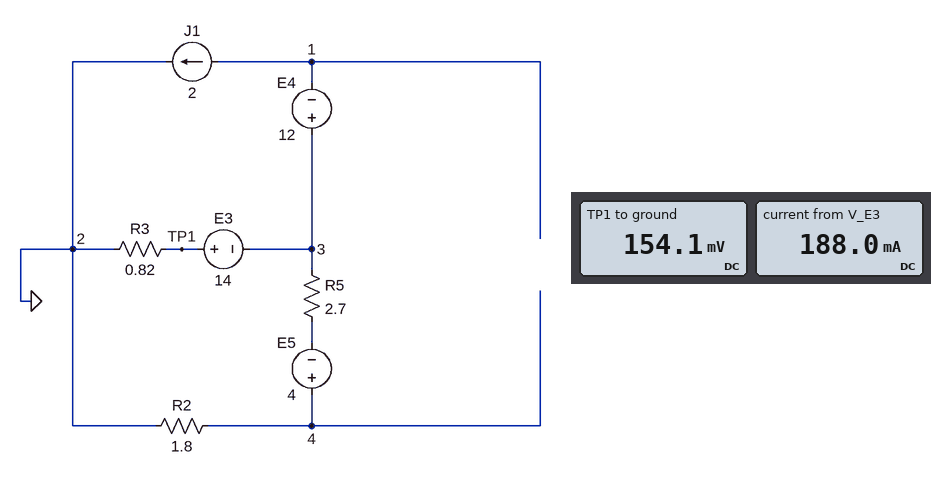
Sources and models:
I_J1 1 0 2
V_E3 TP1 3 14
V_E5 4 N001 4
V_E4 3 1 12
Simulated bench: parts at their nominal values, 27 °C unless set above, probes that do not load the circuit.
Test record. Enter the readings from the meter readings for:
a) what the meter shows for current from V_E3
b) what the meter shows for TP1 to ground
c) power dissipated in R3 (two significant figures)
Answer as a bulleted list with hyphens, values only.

- 188.0 mA
- 154.1 mV
- 29 mW
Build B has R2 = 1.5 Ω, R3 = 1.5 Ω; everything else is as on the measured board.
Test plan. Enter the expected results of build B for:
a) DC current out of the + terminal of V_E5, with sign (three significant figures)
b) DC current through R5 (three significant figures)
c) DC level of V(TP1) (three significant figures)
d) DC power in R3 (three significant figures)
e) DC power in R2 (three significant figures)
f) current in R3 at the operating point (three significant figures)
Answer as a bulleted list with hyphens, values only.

- -2.28 A
- 2.28 A
- 421 mV
- 118 mW
- 7.80 W
- 281 mA
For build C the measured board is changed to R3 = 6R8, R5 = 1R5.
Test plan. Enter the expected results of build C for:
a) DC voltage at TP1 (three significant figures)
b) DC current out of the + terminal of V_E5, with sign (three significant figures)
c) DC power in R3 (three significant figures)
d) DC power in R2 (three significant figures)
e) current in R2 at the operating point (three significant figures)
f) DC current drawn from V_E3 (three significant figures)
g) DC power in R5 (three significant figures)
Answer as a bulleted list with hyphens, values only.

- 2.29 V
- -2.34 A
- 771 mW
- 9.83 W
- 2.34 A
- 337 mA
- 8.19 W
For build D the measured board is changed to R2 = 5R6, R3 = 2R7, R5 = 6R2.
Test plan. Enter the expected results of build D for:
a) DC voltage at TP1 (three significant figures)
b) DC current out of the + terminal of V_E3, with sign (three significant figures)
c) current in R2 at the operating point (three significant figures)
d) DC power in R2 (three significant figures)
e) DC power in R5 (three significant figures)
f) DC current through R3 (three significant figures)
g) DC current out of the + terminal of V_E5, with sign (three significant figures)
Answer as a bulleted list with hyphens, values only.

- -2.53 V
- -938 mA
- 1.06 A
- 6.32 W
- 6.99 W
- 938 mA
- -1.06 A
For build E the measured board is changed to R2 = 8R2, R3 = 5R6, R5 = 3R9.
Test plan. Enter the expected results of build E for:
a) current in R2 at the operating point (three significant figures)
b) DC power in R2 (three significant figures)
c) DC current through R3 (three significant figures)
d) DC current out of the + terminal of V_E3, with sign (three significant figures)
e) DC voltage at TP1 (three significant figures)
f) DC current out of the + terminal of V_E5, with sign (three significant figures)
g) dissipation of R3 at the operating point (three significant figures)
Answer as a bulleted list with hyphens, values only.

- 1.20 A
- 11.8 W
- 802 mA
- -802 mA
- -4.49 V
- -1.20 A
- 3.60 W
